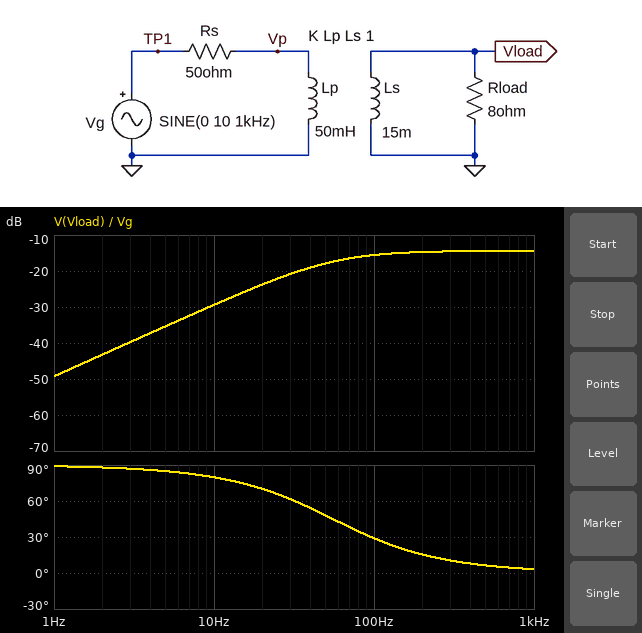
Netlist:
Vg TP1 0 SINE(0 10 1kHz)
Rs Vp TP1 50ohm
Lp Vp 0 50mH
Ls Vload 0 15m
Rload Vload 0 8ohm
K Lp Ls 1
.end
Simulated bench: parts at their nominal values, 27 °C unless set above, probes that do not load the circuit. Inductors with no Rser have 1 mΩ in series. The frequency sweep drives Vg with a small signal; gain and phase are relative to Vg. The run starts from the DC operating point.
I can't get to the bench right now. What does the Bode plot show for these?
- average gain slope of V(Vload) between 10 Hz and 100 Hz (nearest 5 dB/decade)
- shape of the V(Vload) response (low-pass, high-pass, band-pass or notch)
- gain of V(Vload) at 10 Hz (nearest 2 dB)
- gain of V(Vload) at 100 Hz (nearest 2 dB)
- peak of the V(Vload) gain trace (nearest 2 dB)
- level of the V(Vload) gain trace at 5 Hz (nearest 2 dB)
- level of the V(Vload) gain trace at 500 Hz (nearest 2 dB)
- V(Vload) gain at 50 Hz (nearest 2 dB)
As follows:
15 dB/decade
high-pass
-30 dB
-16 dB
-14 dB
-36 dB
-14 dB
-18 dB
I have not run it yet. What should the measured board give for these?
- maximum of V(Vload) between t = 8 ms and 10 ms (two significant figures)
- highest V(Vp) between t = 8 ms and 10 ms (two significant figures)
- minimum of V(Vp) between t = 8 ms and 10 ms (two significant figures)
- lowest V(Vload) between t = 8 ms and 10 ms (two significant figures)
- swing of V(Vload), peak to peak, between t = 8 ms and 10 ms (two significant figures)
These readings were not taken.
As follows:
1.9 V
3.5 V
-3.5 V
-1.9 V
3.8 V
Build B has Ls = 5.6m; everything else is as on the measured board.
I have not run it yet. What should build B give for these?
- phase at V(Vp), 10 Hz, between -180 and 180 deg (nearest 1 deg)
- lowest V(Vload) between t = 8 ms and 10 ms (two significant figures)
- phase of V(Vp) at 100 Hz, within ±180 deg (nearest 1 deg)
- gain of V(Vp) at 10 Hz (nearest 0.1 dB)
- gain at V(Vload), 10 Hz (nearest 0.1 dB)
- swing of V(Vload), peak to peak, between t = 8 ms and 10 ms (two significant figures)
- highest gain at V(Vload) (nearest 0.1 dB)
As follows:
84 deg
-2.0 V
43 deg
-24.1 dB
-33.6 dB
3.9 V
-14.1 dB
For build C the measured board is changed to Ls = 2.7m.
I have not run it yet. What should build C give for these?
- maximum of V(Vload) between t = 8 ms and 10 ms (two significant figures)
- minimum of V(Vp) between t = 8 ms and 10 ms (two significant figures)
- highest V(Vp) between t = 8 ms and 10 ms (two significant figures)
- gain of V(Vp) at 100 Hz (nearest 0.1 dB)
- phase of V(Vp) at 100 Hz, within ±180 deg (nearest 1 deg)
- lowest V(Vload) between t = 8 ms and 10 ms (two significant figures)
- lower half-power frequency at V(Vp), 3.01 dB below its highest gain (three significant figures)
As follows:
1.7 V
-7.4 V
7.4 V
-6.4 dB
50 deg
-1.7 V
119 Hz
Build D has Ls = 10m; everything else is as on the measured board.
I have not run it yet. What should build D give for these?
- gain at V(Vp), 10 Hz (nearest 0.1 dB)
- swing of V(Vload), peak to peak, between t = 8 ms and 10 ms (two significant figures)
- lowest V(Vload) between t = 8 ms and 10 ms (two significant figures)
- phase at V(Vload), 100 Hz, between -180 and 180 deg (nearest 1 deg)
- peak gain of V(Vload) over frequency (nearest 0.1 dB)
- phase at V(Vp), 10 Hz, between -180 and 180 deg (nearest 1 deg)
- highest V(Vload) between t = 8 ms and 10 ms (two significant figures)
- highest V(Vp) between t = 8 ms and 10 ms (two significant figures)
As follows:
-24.1 dB
4.0 V
-2.0 V
35 deg
-14.0 dB
82 deg
2.0 V
4.4 V
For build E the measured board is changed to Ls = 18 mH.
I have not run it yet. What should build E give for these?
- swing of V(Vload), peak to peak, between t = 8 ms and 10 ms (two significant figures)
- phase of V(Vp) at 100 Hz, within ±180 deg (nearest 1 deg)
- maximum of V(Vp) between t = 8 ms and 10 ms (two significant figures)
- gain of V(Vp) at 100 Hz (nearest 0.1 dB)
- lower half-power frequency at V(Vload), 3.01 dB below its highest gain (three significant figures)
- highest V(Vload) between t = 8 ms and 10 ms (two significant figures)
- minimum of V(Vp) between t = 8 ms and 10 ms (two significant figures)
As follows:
3.7 V
26 deg
3.1 V
-11.2 dB
49.0 Hz
1.8 V
-3.1 V
